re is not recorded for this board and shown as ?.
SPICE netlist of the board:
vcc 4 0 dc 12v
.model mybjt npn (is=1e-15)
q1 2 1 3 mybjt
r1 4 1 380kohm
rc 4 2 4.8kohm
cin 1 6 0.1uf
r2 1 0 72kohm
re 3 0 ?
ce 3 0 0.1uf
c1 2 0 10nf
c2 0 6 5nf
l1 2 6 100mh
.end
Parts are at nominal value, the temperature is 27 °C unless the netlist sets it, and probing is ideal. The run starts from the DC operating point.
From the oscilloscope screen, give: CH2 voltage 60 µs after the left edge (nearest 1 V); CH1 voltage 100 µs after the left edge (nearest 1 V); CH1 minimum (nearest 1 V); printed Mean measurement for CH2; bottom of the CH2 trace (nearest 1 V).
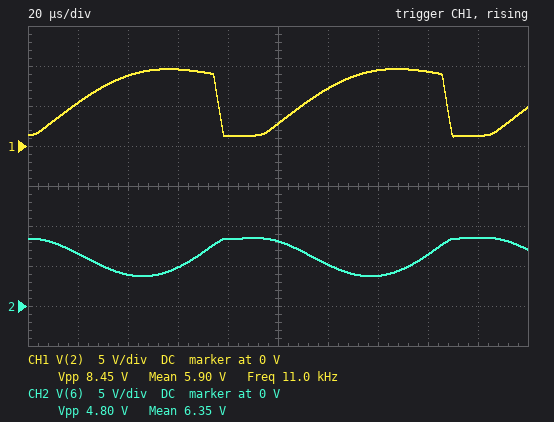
5 V
3 V
1 V
6.35 V
4 V
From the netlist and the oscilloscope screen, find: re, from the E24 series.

680 Ω
